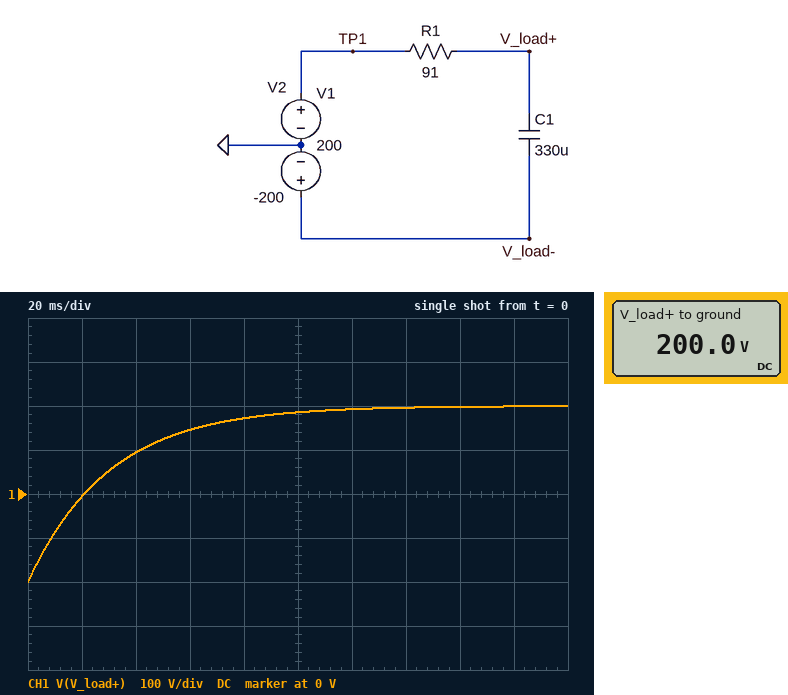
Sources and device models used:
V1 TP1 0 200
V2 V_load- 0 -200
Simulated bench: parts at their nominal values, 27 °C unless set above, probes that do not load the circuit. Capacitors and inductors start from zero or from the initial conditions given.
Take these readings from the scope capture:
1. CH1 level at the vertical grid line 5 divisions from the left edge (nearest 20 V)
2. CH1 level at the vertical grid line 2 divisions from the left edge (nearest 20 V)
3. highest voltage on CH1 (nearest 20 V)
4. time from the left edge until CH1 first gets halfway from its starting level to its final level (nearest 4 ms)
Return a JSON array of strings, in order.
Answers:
["180 V", "100 V", "200 V", "20 ms"]
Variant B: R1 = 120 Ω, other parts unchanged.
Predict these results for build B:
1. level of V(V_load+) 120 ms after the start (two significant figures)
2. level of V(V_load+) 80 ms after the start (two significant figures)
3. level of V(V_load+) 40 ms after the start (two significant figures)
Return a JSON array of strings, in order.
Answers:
["180 V", "150 V", "54 V"]
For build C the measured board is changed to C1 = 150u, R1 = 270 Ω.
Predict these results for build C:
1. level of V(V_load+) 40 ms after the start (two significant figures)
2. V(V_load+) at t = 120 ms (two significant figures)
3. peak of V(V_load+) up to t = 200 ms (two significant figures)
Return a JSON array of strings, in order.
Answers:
["51 V", "180 V", "200 V"]
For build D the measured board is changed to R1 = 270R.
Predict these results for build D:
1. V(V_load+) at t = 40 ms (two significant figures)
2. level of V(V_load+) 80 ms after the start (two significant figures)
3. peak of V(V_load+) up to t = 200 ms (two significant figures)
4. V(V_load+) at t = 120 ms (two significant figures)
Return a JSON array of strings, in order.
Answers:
["-55 V", "37 V", "160 V", "96 V"]
